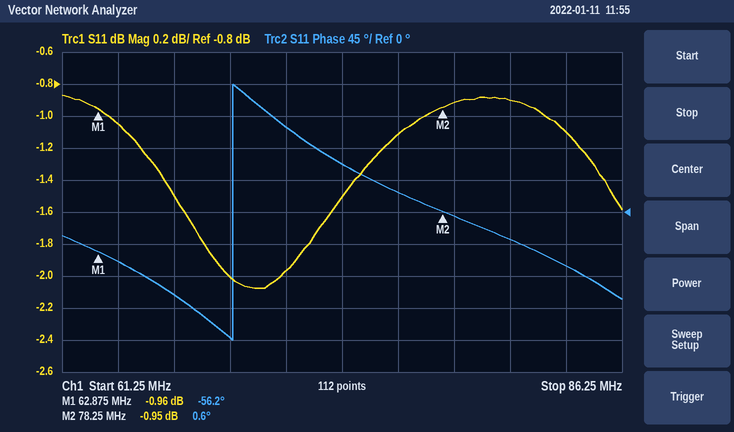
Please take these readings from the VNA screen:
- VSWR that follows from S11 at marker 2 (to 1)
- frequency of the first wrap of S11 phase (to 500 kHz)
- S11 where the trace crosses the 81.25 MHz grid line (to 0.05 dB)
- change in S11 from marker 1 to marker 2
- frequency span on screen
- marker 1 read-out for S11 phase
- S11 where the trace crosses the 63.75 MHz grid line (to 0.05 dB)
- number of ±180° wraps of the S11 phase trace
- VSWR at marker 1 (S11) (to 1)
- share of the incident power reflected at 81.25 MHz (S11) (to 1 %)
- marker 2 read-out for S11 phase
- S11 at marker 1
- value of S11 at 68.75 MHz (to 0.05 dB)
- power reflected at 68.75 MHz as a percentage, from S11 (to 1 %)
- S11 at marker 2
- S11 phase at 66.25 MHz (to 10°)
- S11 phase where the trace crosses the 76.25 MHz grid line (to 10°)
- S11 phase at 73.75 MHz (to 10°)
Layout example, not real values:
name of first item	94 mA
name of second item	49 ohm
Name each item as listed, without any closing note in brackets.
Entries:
VSWR that follows from S11 at marker 2	18
frequency of the first wrap of S11 phase	69.0 MHz
S11 where the trace crosses the 81.25 MHz grid line	-0.90 dB
change in S11 from marker 1 to marker 2	0.01 dB
frequency span on screen	25 MHz
marker 1 read-out for S11 phase	-56.2°
S11 where the trace crosses the 63.75 MHz grid line	-1.05 dB
number of ±180° wraps of the S11 phase trace	1
VSWR at marker 1 (S11)	18
share of the incident power reflected at 81.25 MHz (S11)	81 %
marker 2 read-out for S11 phase	0.6°
S11 at marker 1	-0.96 dB
value of S11 at 68.75 MHz	-2.00 dB
power reflected at 68.75 MHz as a percentage, from S11	63 %
S11 at marker 2	-0.95 dB
S11 phase at 66.25 MHz	-120°
S11 phase where the trace crosses the 76.25 MHz grid line	30°
S11 phase at 73.75 MHz	70°
